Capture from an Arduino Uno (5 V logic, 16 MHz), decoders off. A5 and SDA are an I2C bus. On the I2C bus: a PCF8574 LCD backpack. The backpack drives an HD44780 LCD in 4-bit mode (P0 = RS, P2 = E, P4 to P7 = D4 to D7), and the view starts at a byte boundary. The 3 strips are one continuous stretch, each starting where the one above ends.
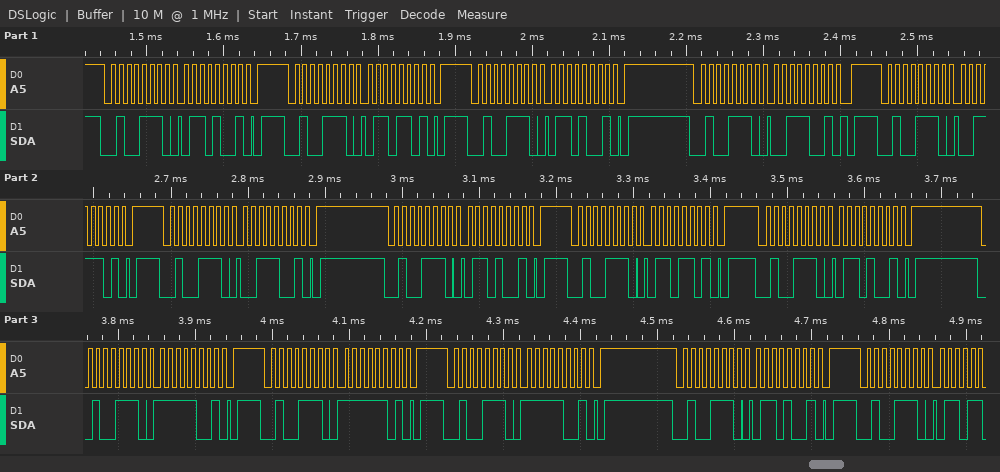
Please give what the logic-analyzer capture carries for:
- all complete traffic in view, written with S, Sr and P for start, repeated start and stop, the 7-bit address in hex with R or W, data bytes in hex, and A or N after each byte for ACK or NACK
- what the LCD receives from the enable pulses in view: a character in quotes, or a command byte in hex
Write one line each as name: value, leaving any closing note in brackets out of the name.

all complete traffic in view, written with S, Sr and P for start, repeated start and stop, the 7-bit address in hex with R or W, data bytes in hex, and A or N after each byte for ACK or NACK: S 27W A 69 A P S 27W A 6D A P S 27W A 69 A P S 27W A 39 A P S 27W A 3D A P S 27W A 39 A P S 27W A 69 A P S 27W A 6D A P S 27W A 69 A P S 27W A F9 A P S 27W A FD A P S 27W A F9 A P S 27W A 69 A P S 27W A
what the LCD receives from the enable pulses in view: a character in quotes, or a command byte in hex: 'c' 'o'
